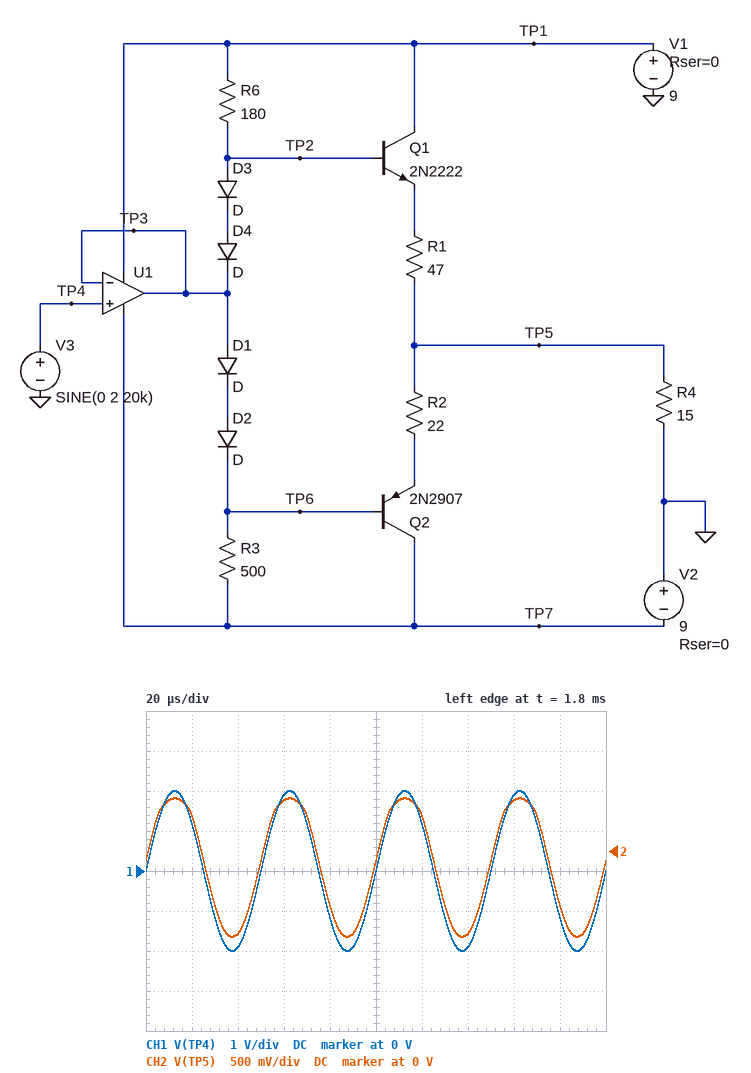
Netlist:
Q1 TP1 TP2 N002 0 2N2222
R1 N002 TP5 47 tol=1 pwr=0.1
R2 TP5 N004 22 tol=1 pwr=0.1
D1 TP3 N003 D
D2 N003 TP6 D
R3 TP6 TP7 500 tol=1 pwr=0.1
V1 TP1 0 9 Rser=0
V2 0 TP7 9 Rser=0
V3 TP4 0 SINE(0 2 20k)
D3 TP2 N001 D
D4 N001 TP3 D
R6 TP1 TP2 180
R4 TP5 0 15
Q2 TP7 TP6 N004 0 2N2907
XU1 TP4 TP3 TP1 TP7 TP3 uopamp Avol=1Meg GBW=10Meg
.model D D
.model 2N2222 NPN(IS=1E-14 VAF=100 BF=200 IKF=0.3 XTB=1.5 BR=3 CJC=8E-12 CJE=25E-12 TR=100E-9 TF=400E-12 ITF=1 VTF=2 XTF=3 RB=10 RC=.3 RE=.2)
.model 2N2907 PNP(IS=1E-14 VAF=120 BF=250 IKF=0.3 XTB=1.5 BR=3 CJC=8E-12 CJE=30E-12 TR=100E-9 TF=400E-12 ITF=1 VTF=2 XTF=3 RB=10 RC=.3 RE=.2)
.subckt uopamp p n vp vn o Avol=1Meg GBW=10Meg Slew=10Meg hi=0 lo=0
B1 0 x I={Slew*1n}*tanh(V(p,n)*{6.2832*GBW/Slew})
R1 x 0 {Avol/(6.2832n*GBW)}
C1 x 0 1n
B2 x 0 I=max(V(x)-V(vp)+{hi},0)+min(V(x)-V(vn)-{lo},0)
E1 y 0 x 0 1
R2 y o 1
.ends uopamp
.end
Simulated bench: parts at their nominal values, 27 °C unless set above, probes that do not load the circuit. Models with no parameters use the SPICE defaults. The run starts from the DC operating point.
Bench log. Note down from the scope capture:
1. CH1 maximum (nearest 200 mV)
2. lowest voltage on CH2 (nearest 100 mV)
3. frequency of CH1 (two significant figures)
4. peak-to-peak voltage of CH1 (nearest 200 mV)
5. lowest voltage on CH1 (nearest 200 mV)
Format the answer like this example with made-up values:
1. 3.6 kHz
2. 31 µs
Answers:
1. 2.0 V
2. -1.1 V
3. 20 kHz
4. 4.0 V
5. -2.0 V
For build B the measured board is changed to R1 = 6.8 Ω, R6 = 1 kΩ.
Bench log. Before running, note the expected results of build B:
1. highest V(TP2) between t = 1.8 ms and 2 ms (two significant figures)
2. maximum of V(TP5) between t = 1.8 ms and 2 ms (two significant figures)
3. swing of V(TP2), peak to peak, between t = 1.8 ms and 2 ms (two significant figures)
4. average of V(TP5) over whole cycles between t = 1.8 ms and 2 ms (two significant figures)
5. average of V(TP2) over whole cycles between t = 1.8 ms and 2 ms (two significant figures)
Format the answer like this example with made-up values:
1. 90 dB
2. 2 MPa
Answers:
1. 3.4 V
2. 1.7 V
3. 4.0 V
4. 260 mV
5. 1.4 V
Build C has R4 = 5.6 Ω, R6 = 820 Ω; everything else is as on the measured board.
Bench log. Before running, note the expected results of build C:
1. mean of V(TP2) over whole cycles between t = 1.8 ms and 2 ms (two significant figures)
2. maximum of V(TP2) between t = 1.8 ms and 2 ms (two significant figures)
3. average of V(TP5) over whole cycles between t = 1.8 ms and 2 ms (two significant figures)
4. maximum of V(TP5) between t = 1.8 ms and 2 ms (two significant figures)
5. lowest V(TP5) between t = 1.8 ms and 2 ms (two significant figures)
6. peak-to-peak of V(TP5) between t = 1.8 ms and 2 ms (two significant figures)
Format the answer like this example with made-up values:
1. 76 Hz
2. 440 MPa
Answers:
1. 1.4 V
2. 3.4 V
3. -97 mV
4. 280 mV
5. -530 mV
6. 810 mV
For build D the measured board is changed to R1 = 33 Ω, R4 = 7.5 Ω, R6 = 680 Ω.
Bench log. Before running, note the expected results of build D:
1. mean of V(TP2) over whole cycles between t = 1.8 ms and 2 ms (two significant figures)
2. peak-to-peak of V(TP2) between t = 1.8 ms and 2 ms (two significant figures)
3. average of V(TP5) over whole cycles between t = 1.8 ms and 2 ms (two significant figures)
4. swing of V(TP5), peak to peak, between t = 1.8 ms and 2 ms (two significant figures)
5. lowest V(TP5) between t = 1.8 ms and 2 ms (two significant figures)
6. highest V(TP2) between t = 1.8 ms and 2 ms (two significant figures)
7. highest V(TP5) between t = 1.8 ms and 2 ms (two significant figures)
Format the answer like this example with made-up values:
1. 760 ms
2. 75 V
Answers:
1. 1.4 V
2. 4.0 V
3. -70 mV
4. 1.2 V
5. -670 mV
6. 3.4 V
7. 490 mV
